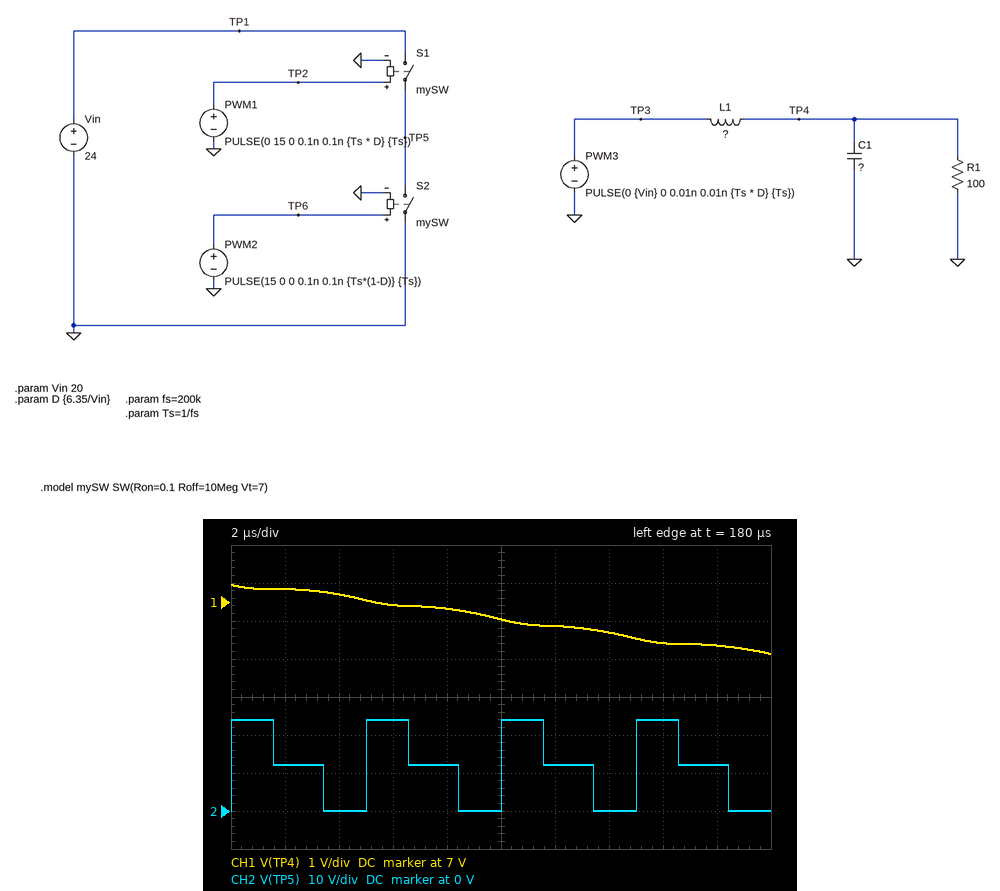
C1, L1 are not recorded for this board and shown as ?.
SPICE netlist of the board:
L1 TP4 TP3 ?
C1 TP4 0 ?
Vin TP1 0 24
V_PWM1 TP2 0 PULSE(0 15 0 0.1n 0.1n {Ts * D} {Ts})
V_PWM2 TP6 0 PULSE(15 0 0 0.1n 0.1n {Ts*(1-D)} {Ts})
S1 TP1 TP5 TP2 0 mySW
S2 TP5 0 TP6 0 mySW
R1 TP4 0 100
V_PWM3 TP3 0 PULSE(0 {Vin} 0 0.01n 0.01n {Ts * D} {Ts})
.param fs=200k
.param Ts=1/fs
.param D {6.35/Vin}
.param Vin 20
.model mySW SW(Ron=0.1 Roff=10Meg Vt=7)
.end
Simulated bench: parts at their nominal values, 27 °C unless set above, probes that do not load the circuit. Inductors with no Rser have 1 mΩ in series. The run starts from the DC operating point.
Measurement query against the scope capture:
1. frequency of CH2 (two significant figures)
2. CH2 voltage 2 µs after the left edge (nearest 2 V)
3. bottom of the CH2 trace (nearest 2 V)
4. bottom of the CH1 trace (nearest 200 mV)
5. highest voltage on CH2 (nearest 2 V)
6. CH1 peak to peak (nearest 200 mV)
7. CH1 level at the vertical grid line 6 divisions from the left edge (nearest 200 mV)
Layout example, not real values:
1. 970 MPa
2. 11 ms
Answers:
1. 200 kHz
2. 12 V
3. 0 V
4. 5.6 V
5. 24 V
6. 1.8 V
7. 6.4 V
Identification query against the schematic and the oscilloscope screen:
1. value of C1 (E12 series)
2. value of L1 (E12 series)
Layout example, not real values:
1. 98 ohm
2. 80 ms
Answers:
1. 560 nF
2. 220 µH
